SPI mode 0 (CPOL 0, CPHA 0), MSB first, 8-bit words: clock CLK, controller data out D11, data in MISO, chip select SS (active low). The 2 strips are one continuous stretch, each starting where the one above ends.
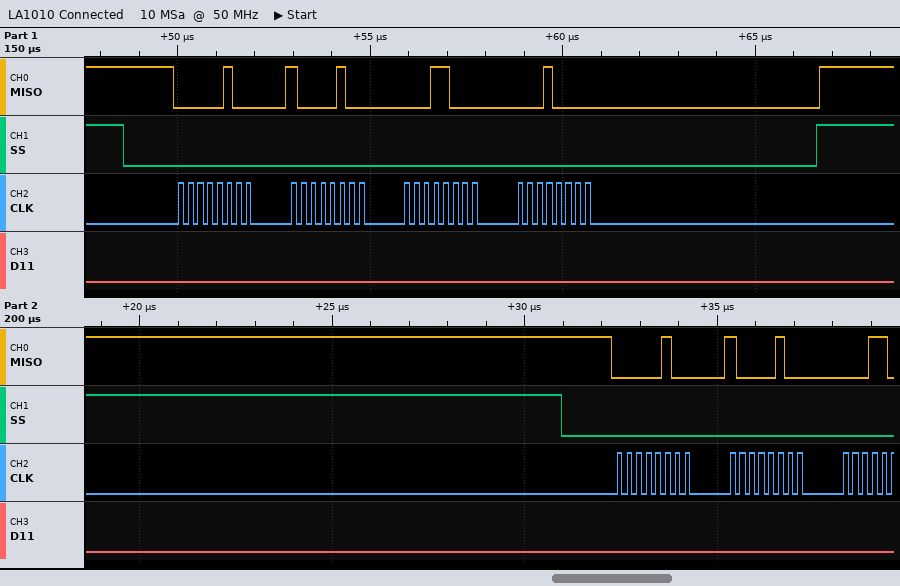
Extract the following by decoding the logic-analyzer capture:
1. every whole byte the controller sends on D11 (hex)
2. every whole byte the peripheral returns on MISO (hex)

0x00 0x00 0x00 0x00 0x00 0x00
0x04 0x84 0x18 0x10 0x04 0x84
